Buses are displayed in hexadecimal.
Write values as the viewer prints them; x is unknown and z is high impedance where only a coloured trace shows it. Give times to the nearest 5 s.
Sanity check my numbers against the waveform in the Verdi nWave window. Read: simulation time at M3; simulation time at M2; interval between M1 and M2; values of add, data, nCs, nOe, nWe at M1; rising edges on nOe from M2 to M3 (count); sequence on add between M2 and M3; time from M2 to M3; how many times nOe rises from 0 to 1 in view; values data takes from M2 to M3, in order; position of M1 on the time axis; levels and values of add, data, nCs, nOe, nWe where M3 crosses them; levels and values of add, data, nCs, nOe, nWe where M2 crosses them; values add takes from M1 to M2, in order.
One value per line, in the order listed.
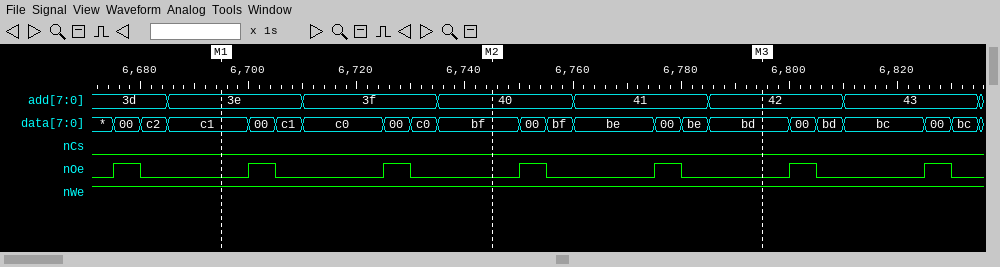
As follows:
6795 s
6745 s
50 s
add=3e, data=c1, nCs=0, nOe=0, nWe=1
2
40, 41, 42
50 s
7
bf, 00, bf, be, 00, be, bd
6695 s
add=42, data=bd, nCs=0, nOe=0, nWe=1
add=40, data=bf, nCs=0, nOe=0, nWe=1
3e, 3f, 40
